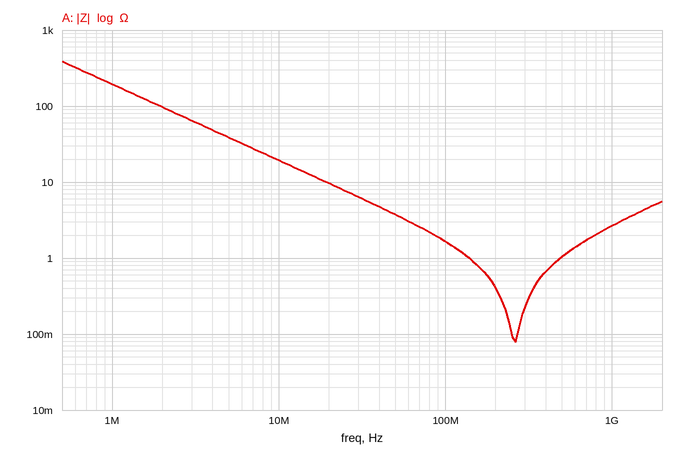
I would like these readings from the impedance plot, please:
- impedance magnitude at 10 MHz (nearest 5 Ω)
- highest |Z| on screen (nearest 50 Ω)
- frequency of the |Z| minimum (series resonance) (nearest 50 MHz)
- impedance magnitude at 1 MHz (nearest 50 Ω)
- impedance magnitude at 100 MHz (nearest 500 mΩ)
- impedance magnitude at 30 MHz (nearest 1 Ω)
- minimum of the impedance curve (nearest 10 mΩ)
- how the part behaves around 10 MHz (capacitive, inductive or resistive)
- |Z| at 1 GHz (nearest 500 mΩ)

20 Ω
400 Ω
250 MHz
200 Ω
1.5 Ω
6 Ω
80 mΩ
capacitive
2.5 Ω
